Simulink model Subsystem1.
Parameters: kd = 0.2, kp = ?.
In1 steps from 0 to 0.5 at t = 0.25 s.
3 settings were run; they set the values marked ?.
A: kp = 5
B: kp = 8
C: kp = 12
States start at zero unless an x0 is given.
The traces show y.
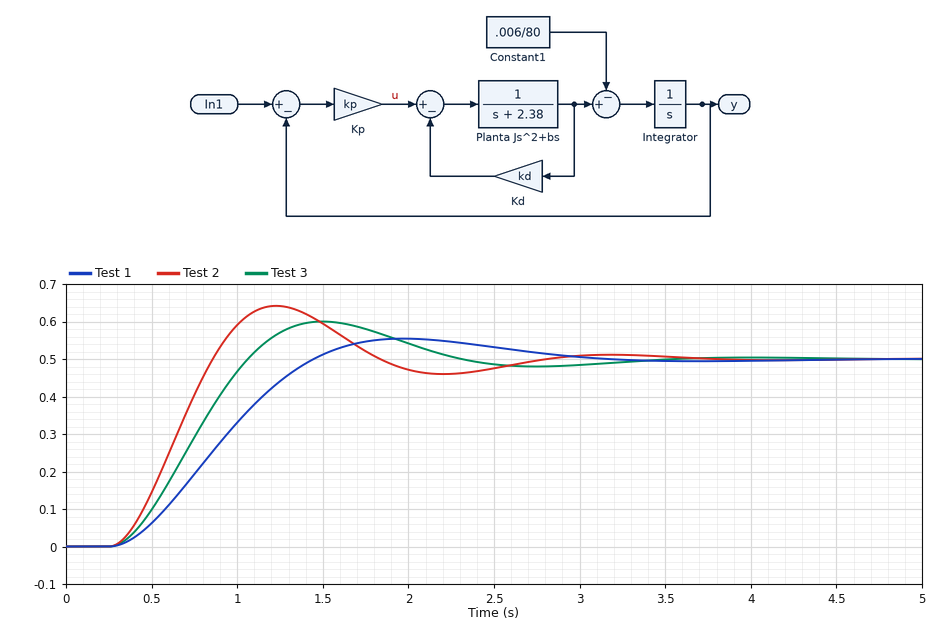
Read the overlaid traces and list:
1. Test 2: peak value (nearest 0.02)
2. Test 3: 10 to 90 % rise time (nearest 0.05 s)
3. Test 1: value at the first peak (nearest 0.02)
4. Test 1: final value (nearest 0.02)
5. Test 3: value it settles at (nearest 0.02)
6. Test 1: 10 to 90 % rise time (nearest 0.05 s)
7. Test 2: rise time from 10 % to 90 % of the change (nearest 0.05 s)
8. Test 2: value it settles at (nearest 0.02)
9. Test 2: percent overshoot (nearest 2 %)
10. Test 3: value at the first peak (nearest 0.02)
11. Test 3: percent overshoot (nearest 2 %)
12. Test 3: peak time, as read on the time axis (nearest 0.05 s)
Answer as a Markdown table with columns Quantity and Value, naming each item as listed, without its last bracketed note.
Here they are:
| Quantity | Value |
|---|---|
| Test 2: peak value | 0.64 |
| Test 3: 10 to 90 % rise time | 0.55 s |
| Test 1: value at the first peak | 0.56 |
| Test 1: final value | 0.50 |
| Test 3: value it settles at | 0.50 |
| Test 1: 10 to 90 % rise time | 0.80 s |
| Test 2: rise time from 10 % to 90 % of the change | 0.40 s |
| Test 2: value it settles at | 0.50 |
| Test 2: percent overshoot | 28 % |
| Test 3: value at the first peak | 0.60 |
| Test 3: percent overshoot | 20 % |
| Test 3: peak time, as read on the time axis | 1.50 s |
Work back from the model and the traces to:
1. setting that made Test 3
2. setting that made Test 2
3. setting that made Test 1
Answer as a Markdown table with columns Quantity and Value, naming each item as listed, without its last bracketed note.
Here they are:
| Quantity | Value |
|---|---|
| setting that made Test 3 | B |
| setting that made Test 2 | C |
| setting that made Test 1 | A |
